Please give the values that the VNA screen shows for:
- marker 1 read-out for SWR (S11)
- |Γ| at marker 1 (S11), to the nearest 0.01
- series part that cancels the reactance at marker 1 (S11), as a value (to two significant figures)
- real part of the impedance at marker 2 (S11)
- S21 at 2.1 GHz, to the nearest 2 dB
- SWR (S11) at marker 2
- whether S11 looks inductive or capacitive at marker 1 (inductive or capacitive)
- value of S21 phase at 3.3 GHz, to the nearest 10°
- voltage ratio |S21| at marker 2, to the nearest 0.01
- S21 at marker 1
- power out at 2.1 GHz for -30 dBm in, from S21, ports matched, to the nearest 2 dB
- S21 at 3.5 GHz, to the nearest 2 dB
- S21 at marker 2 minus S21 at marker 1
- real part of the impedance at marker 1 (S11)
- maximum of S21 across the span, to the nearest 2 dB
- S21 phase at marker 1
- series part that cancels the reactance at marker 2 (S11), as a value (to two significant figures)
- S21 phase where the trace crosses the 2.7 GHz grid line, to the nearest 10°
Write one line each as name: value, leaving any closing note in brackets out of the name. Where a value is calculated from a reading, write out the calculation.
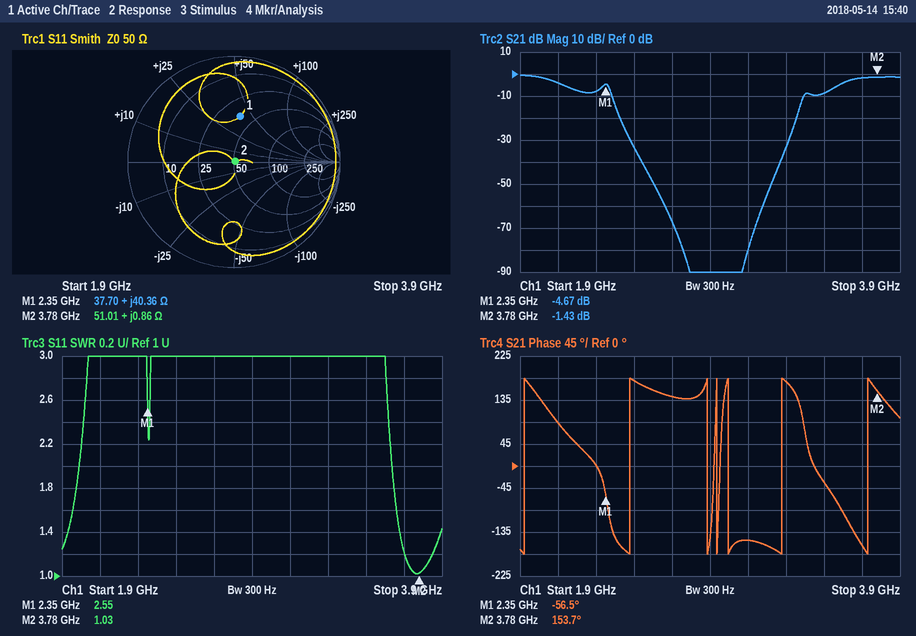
marker 1 read-out for SWR: 2.55
|Γ| at marker 1 (S11), to the nearest 0.01: 0.44
series part that cancels the reactance at marker 1 (S11), as a value: C = 1/(2π × 2.35 GHz × 40.36 Ω) ≈ 1.7 pF
real part of the impedance at marker 2: 51.01 Ω
S21 at 2.1 GHz, to the nearest 2 dB: -4 dB
SWR (S11) at marker 2: 1.03
whether S11 looks inductive or capacitive at marker 1: inductive
value of S21 phase at 3.3 GHz, to the nearest 10°: 170°
voltage ratio |S21| at marker 2, to the nearest 0.01: 10^(-1.43/20) ≈ 0.85
S21 at marker 1: -4.67 dB
power out at 2.1 GHz for -30 dBm in, from S21, ports matched, to the nearest 2 dB: -30 dBm + (-4 dB) = -34 dBm
S21 at 3.5 GHz, to the nearest 2 dB: -8 dB
S21 at marker 2 minus S21 at marker 1: -1.43 − (-4.67) = 3.24 dB
real part of the impedance at marker 1: 37.70 Ω
maximum of S21 across the span, to the nearest 2 dB: 0 dB
S21 phase at marker 1: -56.5°
series part that cancels the reactance at marker 2 (S11), as a value: C = 1/(2π × 3.78 GHz × 0.86 Ω) ≈ 49 pF
S21 phase where the trace crosses the 2.7 GHz grid line, to the nearest 10°: 140°
